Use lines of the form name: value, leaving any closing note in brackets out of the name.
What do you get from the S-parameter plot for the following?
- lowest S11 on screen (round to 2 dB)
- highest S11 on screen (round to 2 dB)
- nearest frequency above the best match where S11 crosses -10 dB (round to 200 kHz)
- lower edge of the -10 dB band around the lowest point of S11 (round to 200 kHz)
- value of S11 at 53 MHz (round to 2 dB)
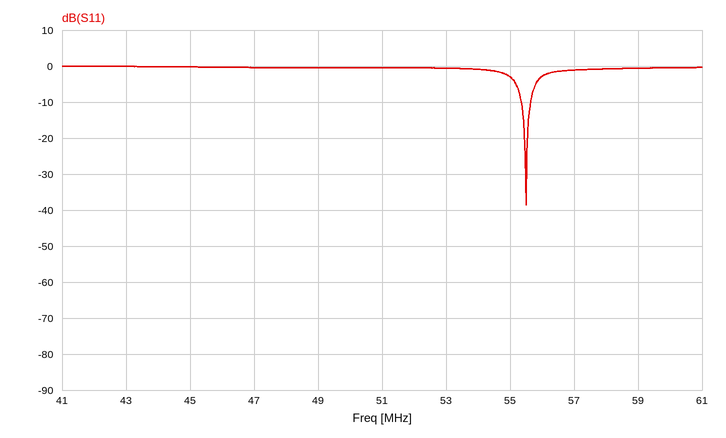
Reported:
lowest S11 on screen: -38 dB
highest S11 on screen: 0 dB
nearest frequency above the best match where S11 crosses -10 dB: 55.6 MHz
lower edge of the -10 dB band around the lowest point of S11: 55.4 MHz
value of S11 at 53 MHz: 0 dB
